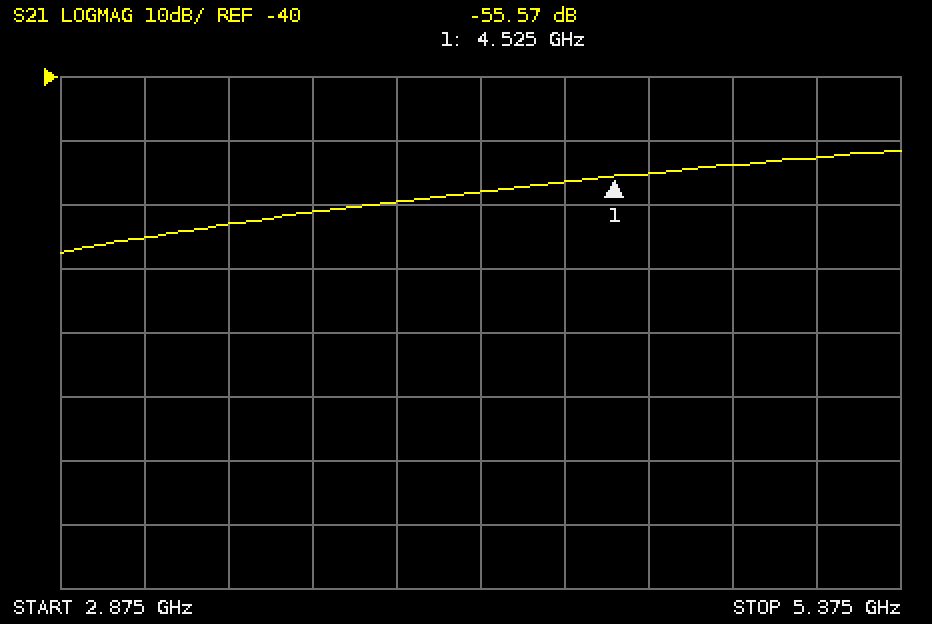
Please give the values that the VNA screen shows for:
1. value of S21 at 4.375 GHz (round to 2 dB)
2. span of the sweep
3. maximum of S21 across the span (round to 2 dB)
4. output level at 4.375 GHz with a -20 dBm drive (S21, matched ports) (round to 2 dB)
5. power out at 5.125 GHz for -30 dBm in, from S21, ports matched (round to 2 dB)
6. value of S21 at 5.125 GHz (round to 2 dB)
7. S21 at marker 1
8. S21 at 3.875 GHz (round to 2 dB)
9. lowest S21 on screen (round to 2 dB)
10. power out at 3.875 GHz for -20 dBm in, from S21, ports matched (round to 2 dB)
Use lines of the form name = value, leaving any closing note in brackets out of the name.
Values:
value of S21 at 4.375 GHz = -56 dB
span of the sweep = 2.5 GHz
maximum of S21 across the span = -52 dB
output level at 4.375 GHz with a -20 dBm drive (S21, matched ports) = -76 dBm
power out at 5.125 GHz for -30 dBm in, from S21, ports matched = -82 dBm
value of S21 at 5.125 GHz = -52 dB
S21 at marker 1 = -55.57 dB
S21 at 3.875 GHz = -60 dB
lowest S21 on screen = -68 dB
power out at 3.875 GHz for -20 dBm in, from S21, ports matched = -80 dBm
